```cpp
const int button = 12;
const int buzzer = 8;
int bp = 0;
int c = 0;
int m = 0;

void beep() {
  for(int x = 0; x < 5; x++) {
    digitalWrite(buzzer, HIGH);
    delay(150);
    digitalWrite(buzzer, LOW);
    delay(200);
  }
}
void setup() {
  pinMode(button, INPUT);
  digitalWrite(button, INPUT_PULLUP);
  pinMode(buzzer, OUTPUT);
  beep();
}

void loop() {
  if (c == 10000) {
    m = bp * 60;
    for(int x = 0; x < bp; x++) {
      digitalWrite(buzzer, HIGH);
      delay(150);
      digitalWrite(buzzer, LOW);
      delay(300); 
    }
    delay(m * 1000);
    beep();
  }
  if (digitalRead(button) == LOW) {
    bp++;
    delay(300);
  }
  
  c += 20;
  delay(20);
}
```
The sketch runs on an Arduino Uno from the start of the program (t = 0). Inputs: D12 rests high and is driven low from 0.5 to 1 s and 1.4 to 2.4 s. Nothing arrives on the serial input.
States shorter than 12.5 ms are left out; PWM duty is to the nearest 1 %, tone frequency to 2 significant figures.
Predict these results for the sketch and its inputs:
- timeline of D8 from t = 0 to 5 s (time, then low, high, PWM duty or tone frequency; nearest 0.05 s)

0 s high; 0.15 s low; 0.35 s high; 0.5 s low; 0.7 s high; 0.85 s low; 1.05 s high; 1.2 s low; 1.4 s high; 1.55 s low
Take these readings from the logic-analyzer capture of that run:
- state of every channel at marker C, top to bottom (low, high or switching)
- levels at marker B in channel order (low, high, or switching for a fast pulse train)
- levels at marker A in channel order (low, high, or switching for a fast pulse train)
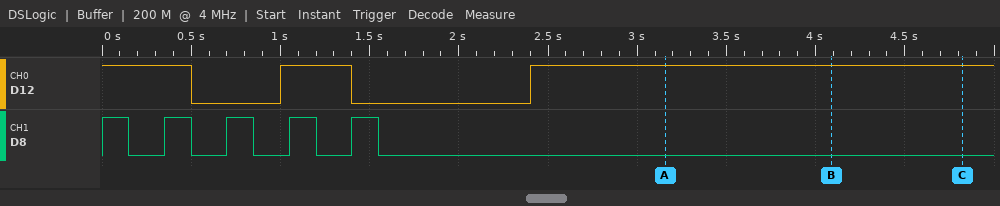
D12 high, D8 low
D12 high, D8 low
D12 high, D8 low
